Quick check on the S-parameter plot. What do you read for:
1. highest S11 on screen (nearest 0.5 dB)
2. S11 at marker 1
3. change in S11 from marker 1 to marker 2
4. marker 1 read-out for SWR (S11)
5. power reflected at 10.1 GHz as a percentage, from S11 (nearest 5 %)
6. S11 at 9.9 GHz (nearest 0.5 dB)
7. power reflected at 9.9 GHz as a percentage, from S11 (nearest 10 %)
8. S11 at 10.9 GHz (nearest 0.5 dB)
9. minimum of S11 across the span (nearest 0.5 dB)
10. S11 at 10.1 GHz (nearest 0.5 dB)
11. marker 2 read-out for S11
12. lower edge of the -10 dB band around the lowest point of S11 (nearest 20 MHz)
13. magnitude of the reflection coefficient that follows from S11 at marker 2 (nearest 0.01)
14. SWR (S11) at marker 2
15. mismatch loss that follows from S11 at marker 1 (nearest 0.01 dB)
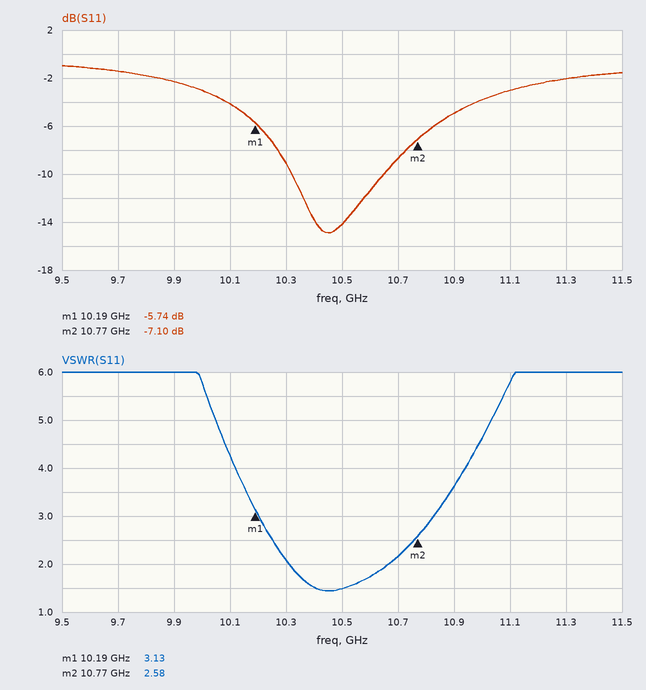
-1.0 dB
-5.74 dB
-1.36 dB
3.13
40 %
-2.5 dB
60 %
-5.0 dB
-15.0 dB
-4.0 dB
-7.10 dB
10.32 GHz
0.44
2.58
1.35 dB
